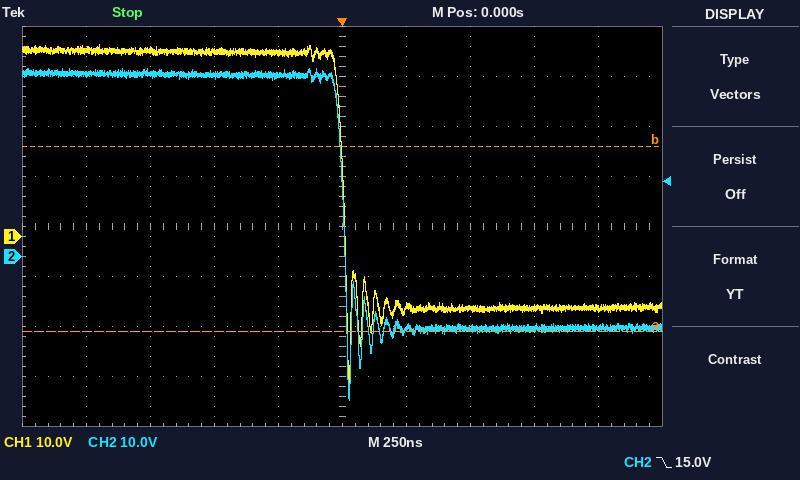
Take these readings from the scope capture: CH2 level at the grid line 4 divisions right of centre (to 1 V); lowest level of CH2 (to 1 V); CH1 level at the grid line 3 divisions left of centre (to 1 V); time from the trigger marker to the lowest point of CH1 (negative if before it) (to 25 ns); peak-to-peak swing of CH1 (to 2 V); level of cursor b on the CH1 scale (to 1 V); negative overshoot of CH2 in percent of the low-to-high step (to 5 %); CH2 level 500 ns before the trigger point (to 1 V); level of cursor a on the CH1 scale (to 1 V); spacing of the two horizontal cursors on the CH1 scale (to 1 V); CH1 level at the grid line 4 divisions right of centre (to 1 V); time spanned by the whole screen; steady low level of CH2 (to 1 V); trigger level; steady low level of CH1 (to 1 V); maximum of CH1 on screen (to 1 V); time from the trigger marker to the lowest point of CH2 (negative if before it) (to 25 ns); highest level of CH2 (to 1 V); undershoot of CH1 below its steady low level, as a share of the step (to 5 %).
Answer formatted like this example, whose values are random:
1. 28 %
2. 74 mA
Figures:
1. -14 V
2. -29 V
3. 37 V
4. +25 ns
5. 68 V
6. 18 V
7. 30 %
8. 36 V
9. -19 V
10. 37 V
11. -14 V
12. 2.5 µs
13. -14 V
14. 15.0 V
15. -14 V
16. 38 V
17. +25 ns
18. 38 V
19. 30 %
